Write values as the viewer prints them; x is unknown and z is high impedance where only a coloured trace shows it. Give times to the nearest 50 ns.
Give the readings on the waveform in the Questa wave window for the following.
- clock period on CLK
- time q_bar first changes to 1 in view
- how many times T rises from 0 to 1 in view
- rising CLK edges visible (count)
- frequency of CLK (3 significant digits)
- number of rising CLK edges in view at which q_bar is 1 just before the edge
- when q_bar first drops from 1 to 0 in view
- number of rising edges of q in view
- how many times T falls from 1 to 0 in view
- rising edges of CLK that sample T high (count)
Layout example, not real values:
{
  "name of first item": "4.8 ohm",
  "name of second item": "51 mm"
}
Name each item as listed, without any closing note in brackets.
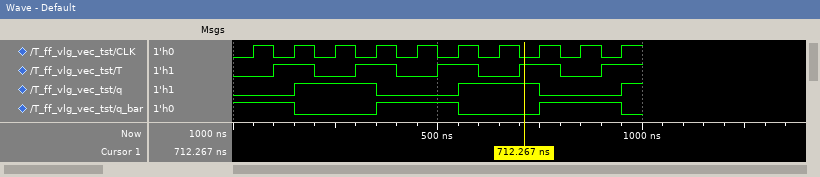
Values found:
{
  "clock period on CLK": "100 ns",
  "time q_bar first changes to 1 in view": "350 ns",
  "how many times T rises from 0 to 1 in view": "5",
  "rising CLK edges visible": "10",
  "frequency of CLK": "10.0 MHz",
  "number of rising CLK edges in view at which q_bar is 1 just before the edge": "6",
  "when q_bar first drops from 1 to 0 in view": "150 ns",
  "number of rising edges of q in view": "3",
  "how many times T falls from 1 to 0 in view": "4",
  "rising edges of CLK that sample T high": "5"
}
